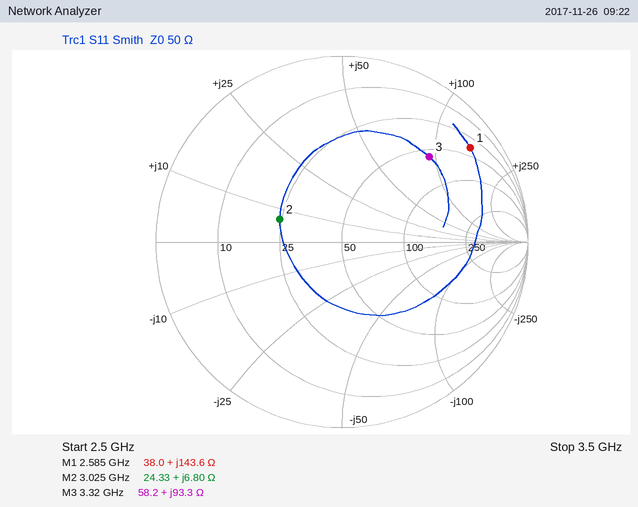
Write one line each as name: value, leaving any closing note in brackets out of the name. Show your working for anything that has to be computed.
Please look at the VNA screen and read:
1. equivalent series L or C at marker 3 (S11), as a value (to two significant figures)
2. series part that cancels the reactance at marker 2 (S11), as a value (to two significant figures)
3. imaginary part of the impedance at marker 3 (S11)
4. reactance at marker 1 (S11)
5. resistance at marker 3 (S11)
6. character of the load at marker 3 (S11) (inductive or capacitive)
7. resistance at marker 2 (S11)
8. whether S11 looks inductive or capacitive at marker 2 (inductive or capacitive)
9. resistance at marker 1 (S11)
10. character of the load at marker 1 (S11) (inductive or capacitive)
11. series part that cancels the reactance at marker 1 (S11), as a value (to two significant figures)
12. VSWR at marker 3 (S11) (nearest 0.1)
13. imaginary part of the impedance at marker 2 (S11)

equivalent series L or C at marker 3 (S11), as a value: L = 93.3 Ω/(2π × 3.32 GHz) ≈ 4.5 nH
series part that cancels the reactance at marker 2 (S11), as a value: C = 1/(2π × 3.025 GHz × 6.8 Ω) ≈ 7.7 pF
imaginary part of the impedance at marker 3: +93.3 Ω
reactance at marker 1: +143.6 Ω
resistance at marker 3: 58.2 Ω
character of the load at marker 3 (S11): inductive
resistance at marker 2: 24.33 Ω
whether S11 looks inductive or capacitive at marker 2: inductive
resistance at marker 1: 38.0 Ω
character of the load at marker 1 (S11): inductive
series part that cancels the reactance at marker 1 (S11), as a value: C = 1/(2π × 2.585 GHz × 143.6 Ω) ≈ 429 fF, so 430 fF to two significant figures
VSWR at marker 3 (S11): 4.8
imaginary part of the impedance at marker 2: +6.80 Ω
